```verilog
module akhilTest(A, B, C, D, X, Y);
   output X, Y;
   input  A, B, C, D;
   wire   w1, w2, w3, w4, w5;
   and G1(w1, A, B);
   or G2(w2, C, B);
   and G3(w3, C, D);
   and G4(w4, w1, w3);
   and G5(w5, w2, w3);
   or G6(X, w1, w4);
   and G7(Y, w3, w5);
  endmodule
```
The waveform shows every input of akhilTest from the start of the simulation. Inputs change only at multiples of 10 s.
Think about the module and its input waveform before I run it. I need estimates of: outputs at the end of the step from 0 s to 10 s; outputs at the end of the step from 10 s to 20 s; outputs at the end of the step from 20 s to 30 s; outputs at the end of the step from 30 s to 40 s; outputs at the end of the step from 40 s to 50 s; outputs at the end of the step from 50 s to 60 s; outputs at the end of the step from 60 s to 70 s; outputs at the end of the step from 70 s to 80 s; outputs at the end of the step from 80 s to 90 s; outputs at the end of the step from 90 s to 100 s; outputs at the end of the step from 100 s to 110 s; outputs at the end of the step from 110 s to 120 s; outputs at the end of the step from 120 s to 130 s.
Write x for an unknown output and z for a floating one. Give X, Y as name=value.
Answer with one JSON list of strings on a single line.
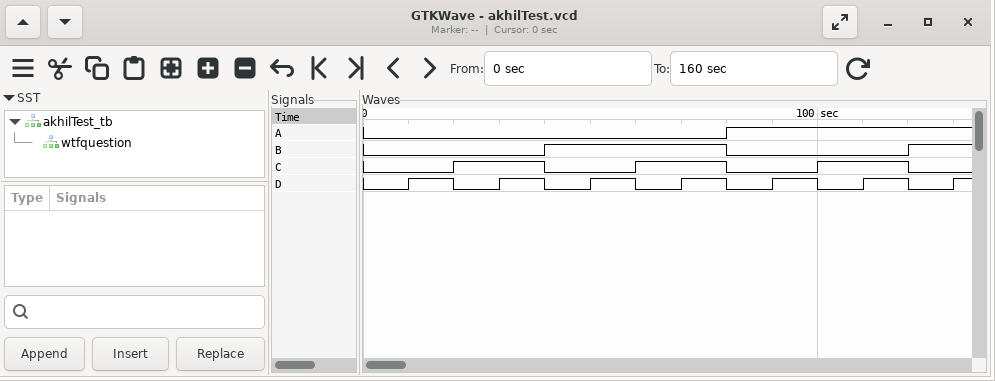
["X=0, Y=0", "X=0, Y=0", "X=0, Y=0", "X=0, Y=1", "X=0, Y=0", "X=0, Y=0", "X=0, Y=0", "X=0, Y=1", "X=0, Y=0", "X=0, Y=0", "X=0, Y=0", "X=0, Y=1", "X=1, Y=0"]
